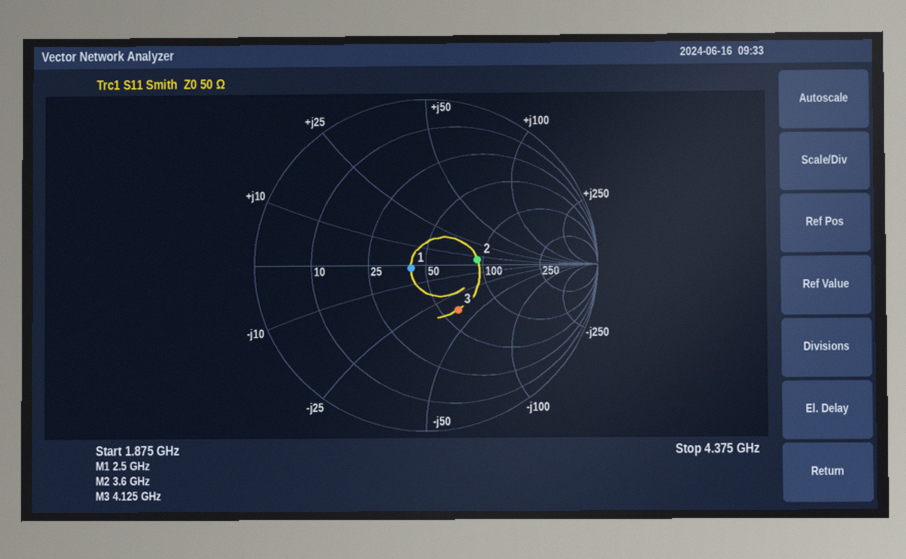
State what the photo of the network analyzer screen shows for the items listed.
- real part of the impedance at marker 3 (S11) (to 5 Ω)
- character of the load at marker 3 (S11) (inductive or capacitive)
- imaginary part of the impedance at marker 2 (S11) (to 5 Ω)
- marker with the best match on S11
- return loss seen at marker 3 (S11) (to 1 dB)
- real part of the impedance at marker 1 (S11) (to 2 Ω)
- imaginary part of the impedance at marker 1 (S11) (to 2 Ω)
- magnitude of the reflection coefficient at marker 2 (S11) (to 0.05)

60 Ω
capacitive
+5 Ω
marker 1
10 dB
42 Ω
-2 Ω
0.30
